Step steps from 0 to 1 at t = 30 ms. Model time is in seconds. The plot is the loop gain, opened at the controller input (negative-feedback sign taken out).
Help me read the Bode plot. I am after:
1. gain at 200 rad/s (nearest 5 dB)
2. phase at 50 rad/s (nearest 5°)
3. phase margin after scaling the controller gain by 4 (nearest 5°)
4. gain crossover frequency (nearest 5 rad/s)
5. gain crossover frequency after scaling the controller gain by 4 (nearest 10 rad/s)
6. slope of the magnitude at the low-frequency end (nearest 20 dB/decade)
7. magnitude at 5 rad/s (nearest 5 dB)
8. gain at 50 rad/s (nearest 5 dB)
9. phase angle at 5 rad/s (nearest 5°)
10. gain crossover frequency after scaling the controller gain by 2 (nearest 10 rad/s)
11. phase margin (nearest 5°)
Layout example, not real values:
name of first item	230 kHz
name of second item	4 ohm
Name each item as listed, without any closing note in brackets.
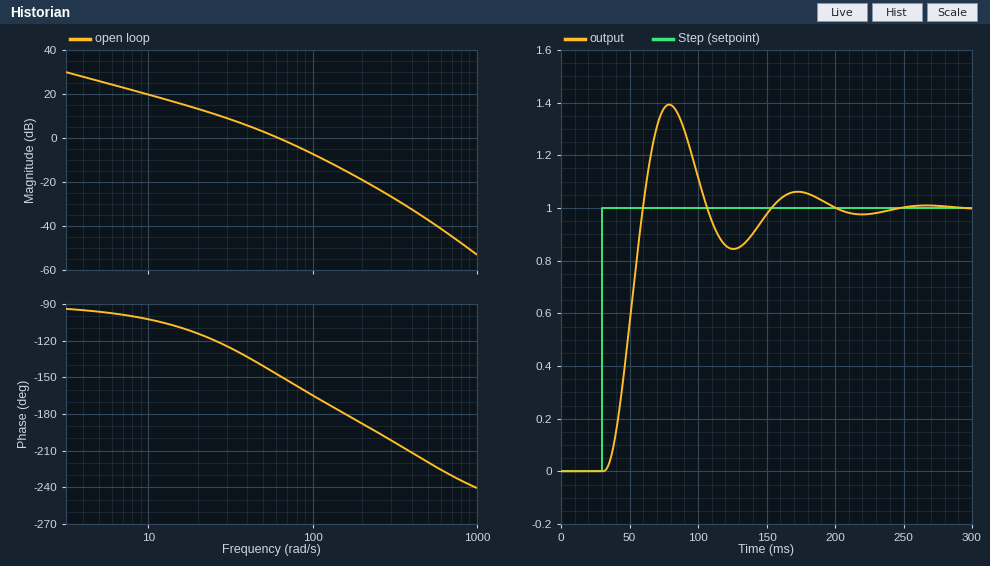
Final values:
gain at 200 rad/s	-20 dB
phase at 50 rad/s	-140°
phase margin after scaling the controller gain by 4	5°
gain crossover frequency	60 rad/s
gain crossover frequency after scaling the controller gain by 4	130 rad/s
slope of the magnitude at the low-frequency end	-20 dB/decade
magnitude at 5 rad/s	25 dB
gain at 50 rad/s	5 dB
phase angle at 5 rad/s	-95°
gain crossover frequency after scaling the controller gain by 2	90 rad/s
phase margin	30°
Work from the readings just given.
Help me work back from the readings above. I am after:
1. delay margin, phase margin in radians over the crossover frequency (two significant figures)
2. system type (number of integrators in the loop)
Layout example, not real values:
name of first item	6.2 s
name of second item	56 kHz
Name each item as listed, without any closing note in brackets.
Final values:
delay margin, phase margin in radians over the crossover frequency	0.0087 s
system type	1
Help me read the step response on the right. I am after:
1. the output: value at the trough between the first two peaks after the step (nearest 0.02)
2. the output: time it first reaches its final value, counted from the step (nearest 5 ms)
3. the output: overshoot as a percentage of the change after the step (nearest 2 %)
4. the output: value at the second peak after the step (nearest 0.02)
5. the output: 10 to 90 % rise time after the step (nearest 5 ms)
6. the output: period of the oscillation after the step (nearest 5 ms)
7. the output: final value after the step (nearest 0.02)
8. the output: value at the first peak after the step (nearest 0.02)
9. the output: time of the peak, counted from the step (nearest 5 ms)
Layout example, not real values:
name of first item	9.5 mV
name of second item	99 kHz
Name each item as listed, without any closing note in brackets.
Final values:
the output: value at the trough between the first two peaks after the step	0.84
the output: time it first reaches its final value, counted from the step	30 ms
the output: overshoot as a percentage of the change after the step	40 %
the output: value at the second peak after the step	1.06
the output: 10 to 90 % rise time after the step	20 ms
the output: period of the oscillation after the step	95 ms
the output: final value after the step	1.00
the output: value at the first peak after the step	1.40
the output: time of the peak, counted from the step	50 ms
